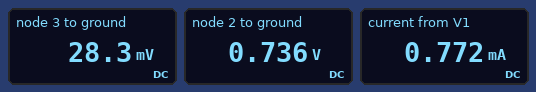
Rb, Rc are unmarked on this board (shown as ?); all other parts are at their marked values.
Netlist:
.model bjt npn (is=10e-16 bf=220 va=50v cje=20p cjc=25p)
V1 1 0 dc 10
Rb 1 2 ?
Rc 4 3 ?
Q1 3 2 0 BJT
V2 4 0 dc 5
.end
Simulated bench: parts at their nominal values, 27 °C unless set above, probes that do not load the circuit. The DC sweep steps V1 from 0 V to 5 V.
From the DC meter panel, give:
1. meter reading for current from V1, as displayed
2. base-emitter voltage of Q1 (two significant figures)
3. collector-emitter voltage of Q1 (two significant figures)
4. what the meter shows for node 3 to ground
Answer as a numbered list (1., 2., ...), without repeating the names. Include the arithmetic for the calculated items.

1. 0.772 mA
2. 736 mV = 740 mV
3. 28.3 mV = 28 mV
4. 28.3 mV
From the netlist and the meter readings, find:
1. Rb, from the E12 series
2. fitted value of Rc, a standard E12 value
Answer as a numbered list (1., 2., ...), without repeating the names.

1. 12 kΩ
2. 6.8 kΩ
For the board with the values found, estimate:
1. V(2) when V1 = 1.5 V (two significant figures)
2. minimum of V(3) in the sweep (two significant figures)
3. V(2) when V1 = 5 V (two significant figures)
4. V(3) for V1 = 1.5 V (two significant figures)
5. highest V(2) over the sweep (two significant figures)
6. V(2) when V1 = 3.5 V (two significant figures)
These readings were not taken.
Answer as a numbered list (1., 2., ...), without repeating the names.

1. 710 mV
2. 37 mV
3. 720 mV
4. 68 mV
5. 720 mV
6. 720 mV
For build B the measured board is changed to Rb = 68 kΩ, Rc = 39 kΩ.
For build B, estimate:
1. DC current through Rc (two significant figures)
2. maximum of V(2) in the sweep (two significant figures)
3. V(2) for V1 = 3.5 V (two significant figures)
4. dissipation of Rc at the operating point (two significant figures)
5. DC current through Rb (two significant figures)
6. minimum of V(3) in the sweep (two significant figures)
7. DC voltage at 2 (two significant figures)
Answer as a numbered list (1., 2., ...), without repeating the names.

1. 130 µA
2. 680 mV
3. 670 mV
4. 630 µW
5. 140 µA
6. 36 mV
7. 690 mV
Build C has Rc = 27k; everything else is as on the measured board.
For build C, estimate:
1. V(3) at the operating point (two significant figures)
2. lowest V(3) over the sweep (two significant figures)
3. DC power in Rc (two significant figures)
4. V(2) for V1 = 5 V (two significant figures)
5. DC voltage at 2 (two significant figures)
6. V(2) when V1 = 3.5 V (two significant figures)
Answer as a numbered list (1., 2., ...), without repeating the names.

1. 21 mV
2. 24 mV
3. 920 µW
4. 710 mV
5. 730 mV
6. 700 mV
